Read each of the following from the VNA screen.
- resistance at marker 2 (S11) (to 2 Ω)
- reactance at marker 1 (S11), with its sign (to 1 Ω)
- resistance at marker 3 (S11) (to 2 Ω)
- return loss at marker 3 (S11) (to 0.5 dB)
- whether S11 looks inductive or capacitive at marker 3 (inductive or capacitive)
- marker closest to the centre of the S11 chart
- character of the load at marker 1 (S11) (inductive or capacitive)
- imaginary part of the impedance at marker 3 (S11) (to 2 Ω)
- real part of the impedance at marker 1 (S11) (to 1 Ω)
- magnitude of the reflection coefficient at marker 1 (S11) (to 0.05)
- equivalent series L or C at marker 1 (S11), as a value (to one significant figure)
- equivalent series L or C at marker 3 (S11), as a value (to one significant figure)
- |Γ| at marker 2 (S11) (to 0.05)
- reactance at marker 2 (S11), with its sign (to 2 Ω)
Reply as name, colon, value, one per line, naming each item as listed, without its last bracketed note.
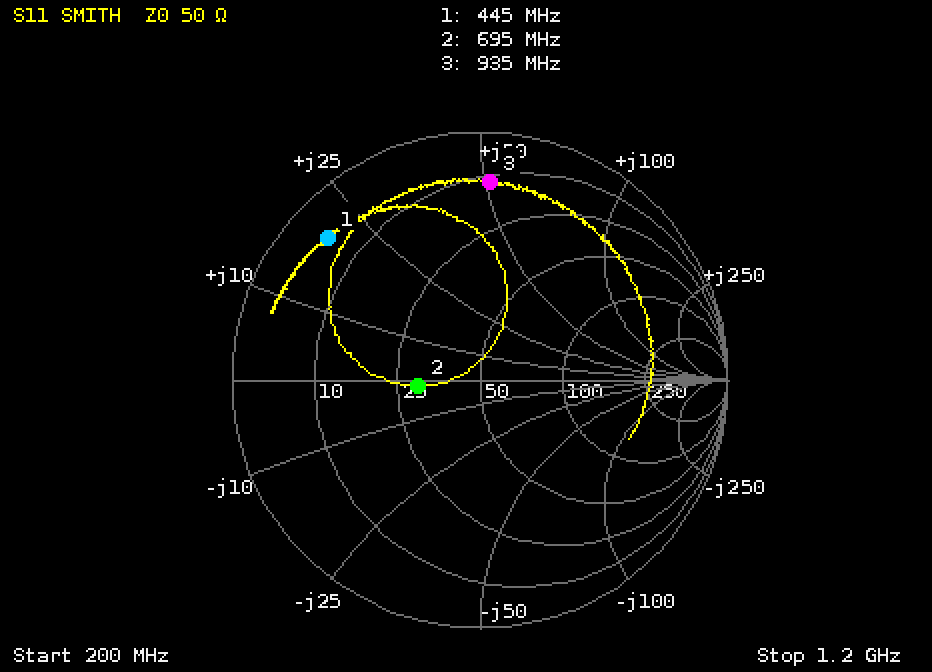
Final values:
resistance at marker 2 (S11): 30 Ω
reactance at marker 1 (S11), with its sign: +20 Ω
resistance at marker 3 (S11): 12 Ω
return loss at marker 3 (S11): 2.0 dB
whether S11 looks inductive or capacitive at marker 3: inductive
marker closest to the centre of the S11 chart: marker 2
character of the load at marker 1 (S11): inductive
imaginary part of the impedance at marker 3 (S11): +52 Ω
real part of the impedance at marker 1 (S11): 5 Ω
magnitude of the reflection coefficient at marker 1 (S11): 0.85
equivalent series L or C at marker 1 (S11), as a value: 7 nH
equivalent series L or C at marker 3 (S11), as a value: 9 nH
|Γ| at marker 2 (S11): 0.25
reactance at marker 2 (S11), with its sign: -2 Ω
